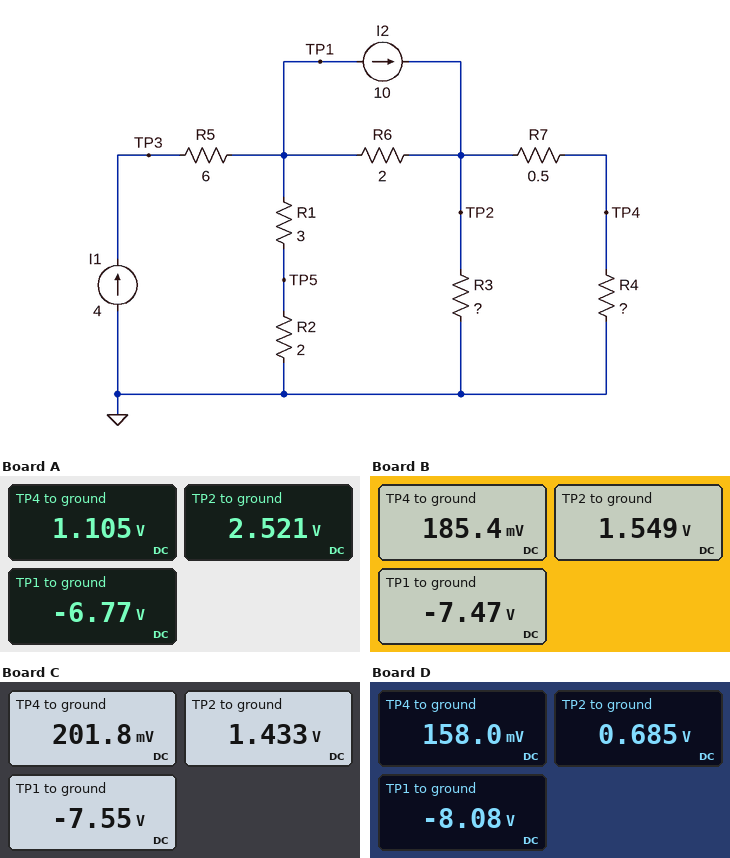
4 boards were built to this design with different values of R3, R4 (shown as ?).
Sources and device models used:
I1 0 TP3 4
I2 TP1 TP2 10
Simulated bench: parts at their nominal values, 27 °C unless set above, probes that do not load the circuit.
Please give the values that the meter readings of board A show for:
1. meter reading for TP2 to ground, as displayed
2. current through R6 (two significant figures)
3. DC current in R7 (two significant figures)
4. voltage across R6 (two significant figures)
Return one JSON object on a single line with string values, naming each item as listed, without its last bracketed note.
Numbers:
{"meter reading for TP2 to ground, as displayed": "2.521 V", "current through R6": "4.6 A", "DC current in R7": "2.8 A", "voltage across R6": "9.3 V"}
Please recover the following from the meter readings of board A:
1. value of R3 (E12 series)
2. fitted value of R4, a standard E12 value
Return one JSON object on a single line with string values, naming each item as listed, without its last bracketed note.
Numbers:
{"value of R3": "1 Ω", "fitted value of R4, a standard E12 value": "0.39 Ω"}
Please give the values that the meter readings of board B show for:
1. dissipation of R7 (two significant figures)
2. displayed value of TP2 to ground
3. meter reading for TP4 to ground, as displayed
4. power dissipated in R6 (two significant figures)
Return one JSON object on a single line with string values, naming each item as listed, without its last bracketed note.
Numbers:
{"dissipation of R7": "3.7 W", "displayed value of TP2 to ground": "1.549 V", "meter reading for TP4 to ground, as displayed": "185.4 mV", "power dissipated in R6": "41 W"}
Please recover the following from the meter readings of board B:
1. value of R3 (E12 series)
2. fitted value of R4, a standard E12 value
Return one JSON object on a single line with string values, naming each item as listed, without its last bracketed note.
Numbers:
{"value of R3": "0.56 Ω", "fitted value of R4, a standard E12 value": "0.068 Ω"}
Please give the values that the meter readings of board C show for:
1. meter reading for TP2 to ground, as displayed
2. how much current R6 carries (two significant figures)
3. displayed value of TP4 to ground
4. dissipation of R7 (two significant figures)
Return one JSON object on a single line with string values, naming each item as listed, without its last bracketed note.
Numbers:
{"meter reading for TP2 to ground, as displayed": "1.433 V", "how much current R6 carries": "4.5 A", "displayed value of TP4 to ground": "201.8 mV", "dissipation of R7": "3.0 W"}
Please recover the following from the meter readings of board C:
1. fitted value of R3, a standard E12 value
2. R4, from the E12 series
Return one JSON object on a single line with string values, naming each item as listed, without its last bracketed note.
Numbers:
{"fitted value of R3, a standard E12 value": "0.47 Ω", "R4, from the E12 series": "0.082 Ω"}
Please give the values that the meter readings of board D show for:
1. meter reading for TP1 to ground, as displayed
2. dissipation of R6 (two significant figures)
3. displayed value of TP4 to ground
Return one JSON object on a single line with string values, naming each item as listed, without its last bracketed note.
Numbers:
{"meter reading for TP1 to ground, as displayed": "-8.08 V", "dissipation of R6": "38 W", "displayed value of TP4 to ground": "158.0 mV"}
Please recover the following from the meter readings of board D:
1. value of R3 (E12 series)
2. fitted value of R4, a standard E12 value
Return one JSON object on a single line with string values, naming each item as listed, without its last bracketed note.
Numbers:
{"value of R3": "0.15 Ω", "fitted value of R4, a standard E12 value": "0.15 Ω"}
